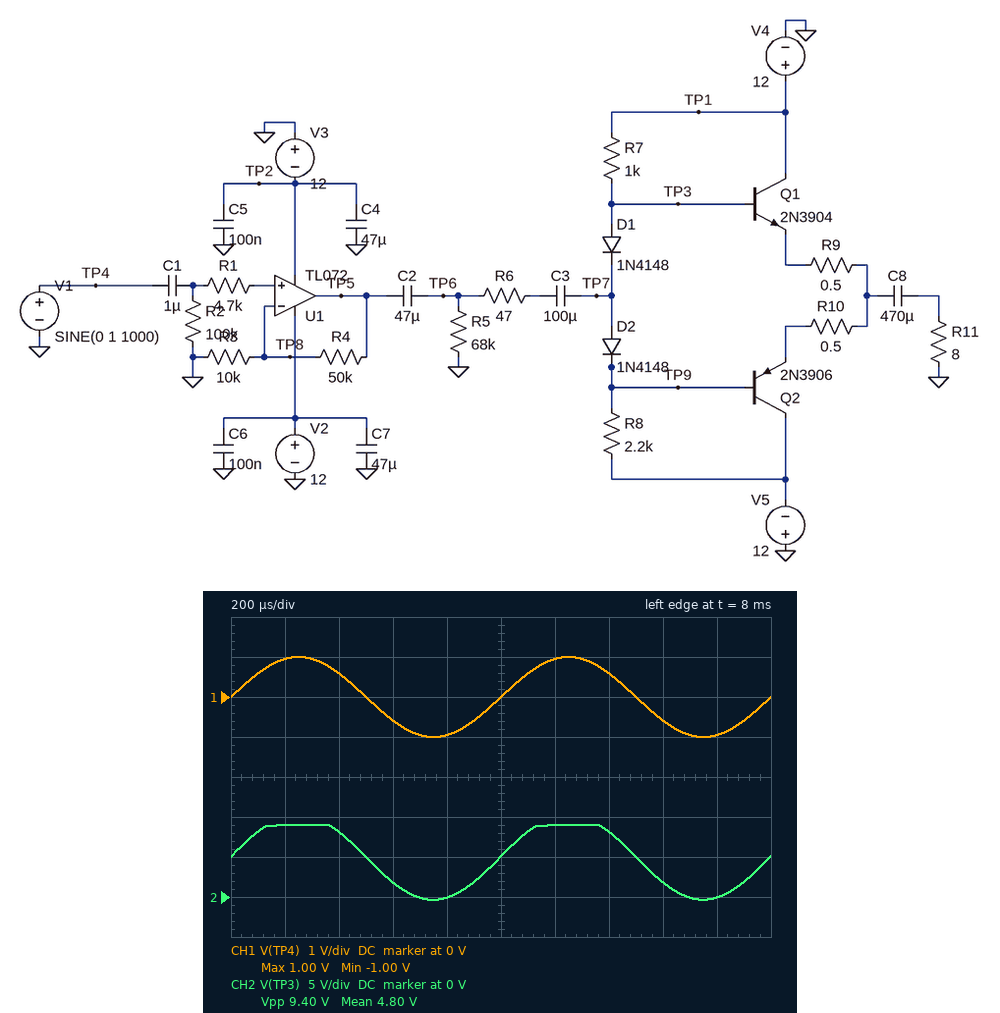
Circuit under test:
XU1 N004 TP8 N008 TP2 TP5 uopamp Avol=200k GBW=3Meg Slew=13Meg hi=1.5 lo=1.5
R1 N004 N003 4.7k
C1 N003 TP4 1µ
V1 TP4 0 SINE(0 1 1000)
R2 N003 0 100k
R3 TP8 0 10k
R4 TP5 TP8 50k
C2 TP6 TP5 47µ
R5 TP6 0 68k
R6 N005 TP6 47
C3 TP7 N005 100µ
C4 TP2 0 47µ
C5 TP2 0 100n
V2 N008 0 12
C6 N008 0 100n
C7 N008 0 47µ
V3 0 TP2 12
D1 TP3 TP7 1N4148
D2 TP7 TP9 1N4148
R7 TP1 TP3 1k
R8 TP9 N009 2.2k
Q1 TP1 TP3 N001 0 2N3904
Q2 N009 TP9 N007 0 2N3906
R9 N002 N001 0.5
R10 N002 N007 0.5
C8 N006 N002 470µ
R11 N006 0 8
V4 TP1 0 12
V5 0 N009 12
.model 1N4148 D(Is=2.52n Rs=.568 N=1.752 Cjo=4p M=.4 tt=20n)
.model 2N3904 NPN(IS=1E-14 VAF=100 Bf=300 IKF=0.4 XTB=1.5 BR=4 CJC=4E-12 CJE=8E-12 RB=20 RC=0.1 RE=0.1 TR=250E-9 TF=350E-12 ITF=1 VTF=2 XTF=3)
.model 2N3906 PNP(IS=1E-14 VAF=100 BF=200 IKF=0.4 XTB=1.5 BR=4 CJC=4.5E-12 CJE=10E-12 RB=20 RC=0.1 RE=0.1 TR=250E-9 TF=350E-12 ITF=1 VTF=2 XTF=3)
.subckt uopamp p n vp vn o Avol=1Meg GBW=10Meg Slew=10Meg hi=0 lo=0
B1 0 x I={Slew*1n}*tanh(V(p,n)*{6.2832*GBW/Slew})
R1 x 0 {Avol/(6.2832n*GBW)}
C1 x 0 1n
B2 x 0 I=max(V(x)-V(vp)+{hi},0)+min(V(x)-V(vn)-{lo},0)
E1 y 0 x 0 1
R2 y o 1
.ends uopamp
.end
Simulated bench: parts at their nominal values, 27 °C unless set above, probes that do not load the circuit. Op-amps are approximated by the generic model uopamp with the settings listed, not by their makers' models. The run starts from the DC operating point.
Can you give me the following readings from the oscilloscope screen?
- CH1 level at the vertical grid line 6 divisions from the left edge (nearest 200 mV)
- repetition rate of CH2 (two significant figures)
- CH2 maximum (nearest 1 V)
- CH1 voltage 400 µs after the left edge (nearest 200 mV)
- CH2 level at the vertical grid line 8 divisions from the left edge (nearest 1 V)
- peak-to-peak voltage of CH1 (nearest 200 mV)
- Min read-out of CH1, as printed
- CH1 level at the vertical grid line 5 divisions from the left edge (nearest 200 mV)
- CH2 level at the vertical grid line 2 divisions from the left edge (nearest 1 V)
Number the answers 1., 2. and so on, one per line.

1. 1.0 V
2. 1.0 kHz
3. 9 V
4. 600 mV
5. 2 V
6. 2.0 V
7. -1.00 V
8. 0 V
9. 8 V
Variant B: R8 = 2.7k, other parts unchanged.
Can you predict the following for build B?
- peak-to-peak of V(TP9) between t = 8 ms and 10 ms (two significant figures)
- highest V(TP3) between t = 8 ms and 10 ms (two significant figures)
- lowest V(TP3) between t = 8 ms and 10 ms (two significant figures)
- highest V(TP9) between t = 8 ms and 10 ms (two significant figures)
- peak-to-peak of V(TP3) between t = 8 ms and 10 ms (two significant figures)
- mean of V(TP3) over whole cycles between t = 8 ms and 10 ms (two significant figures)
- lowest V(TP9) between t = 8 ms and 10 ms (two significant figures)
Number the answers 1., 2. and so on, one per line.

1. 10 V
2. 9.5 V
3. 580 mV
4. 10 V
5. 8.9 V
6. 5.6 V
7. -59 mV
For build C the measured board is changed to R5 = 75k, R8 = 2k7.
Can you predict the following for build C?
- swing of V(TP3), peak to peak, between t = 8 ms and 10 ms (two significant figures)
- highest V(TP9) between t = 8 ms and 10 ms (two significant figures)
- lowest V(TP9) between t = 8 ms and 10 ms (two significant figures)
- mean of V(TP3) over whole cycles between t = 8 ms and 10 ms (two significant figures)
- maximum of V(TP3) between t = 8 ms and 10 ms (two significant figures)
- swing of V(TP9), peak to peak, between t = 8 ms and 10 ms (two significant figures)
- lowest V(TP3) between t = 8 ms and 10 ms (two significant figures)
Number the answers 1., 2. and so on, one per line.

1. 8.9 V
2. 10 V
3. -59 mV
4. 5.6 V
5. 9.5 V
6. 10 V
7. 580 mV
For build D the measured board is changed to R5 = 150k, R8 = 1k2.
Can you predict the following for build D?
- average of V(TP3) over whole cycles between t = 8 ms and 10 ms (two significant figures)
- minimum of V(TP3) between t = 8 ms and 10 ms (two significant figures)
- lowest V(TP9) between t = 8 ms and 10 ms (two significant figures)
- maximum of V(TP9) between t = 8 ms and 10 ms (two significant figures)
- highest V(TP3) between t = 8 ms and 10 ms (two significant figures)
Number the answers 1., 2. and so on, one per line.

1. 1.8 V
2. -3.5 V
3. -4.7 V
4. 5.7 V
5. 7.0 V
